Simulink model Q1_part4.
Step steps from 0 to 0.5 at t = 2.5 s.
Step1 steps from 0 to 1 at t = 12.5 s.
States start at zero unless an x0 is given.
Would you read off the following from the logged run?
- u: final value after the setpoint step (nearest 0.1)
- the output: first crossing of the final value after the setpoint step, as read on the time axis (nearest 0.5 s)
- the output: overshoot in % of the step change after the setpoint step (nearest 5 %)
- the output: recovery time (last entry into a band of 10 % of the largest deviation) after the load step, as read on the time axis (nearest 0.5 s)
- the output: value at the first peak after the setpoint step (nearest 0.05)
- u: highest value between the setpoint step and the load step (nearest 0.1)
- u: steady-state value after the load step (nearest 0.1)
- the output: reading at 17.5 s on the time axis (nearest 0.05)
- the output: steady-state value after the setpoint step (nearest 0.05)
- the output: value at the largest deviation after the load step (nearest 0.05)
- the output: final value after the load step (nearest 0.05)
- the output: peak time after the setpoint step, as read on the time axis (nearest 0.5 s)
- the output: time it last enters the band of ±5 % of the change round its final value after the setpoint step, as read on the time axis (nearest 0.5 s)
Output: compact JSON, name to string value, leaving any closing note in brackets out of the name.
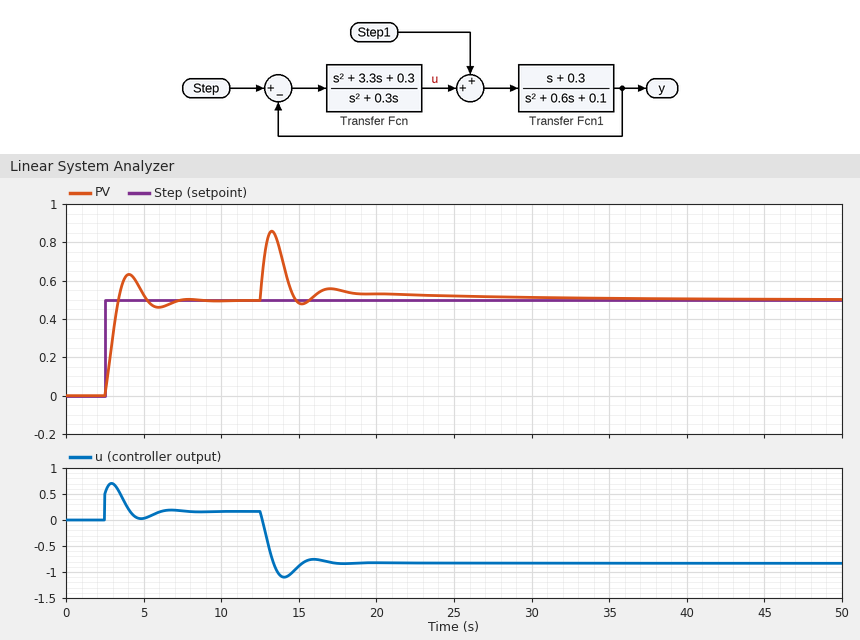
{"u: final value after the setpoint step": "0.2", "the output: first crossing of the final value after the setpoint step, as read on the time axis": "3.5 s", "the output: overshoot in % of the step change after the setpoint step": "25 %", "the output: recovery time (last entry into a band of 10 % of the largest deviation) after the load step, as read on the time axis": "18.5 s", "the output: value at the first peak after the setpoint step": "0.65", "u: highest value between the setpoint step and the load step": "0.7", "u: steady-state value after the load step": "-0.8", "the output: reading at 17.5 s on the time axis": "0.55", "the output: steady-state value after the setpoint step": "0.50", "the output: value at the largest deviation after the load step": "0.85", "the output: final value after the load step": "0.50", "the output: peak time after the setpoint step, as read on the time axis": "4.0 s", "the output: time it last enters the band of ±5 % of the change round its final value after the setpoint step, as read on the time axis": "6.5 s"}
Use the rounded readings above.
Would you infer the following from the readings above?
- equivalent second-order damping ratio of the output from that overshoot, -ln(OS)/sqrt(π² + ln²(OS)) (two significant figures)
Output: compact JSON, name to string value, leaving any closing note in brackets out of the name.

{"equivalent second-order damping ratio of the output from that overshoot, -ln(OS)/sqrt(π² + ln²(OS))": "0.40"}
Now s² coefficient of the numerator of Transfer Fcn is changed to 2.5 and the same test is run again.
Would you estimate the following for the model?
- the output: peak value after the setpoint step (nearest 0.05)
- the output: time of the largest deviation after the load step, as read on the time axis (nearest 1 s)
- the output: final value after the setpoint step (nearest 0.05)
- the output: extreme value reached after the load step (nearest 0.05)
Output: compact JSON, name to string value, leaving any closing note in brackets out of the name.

{"the output: peak value after the setpoint step": "0.55", "the output: time of the largest deviation after the load step, as read on the time axis": "13 s", "the output: final value after the setpoint step": "0.50", "the output: extreme value reached after the load step": "0.75"}
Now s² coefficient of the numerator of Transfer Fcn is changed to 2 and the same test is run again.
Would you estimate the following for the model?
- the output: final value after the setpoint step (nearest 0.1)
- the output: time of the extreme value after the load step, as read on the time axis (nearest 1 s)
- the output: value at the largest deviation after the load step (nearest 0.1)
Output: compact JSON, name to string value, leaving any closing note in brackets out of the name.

{"the output: final value after the setpoint step": "0.5", "the output: time of the extreme value after the load step, as read on the time axis": "13 s", "the output: value at the largest deviation after the load step": "0.8"}
